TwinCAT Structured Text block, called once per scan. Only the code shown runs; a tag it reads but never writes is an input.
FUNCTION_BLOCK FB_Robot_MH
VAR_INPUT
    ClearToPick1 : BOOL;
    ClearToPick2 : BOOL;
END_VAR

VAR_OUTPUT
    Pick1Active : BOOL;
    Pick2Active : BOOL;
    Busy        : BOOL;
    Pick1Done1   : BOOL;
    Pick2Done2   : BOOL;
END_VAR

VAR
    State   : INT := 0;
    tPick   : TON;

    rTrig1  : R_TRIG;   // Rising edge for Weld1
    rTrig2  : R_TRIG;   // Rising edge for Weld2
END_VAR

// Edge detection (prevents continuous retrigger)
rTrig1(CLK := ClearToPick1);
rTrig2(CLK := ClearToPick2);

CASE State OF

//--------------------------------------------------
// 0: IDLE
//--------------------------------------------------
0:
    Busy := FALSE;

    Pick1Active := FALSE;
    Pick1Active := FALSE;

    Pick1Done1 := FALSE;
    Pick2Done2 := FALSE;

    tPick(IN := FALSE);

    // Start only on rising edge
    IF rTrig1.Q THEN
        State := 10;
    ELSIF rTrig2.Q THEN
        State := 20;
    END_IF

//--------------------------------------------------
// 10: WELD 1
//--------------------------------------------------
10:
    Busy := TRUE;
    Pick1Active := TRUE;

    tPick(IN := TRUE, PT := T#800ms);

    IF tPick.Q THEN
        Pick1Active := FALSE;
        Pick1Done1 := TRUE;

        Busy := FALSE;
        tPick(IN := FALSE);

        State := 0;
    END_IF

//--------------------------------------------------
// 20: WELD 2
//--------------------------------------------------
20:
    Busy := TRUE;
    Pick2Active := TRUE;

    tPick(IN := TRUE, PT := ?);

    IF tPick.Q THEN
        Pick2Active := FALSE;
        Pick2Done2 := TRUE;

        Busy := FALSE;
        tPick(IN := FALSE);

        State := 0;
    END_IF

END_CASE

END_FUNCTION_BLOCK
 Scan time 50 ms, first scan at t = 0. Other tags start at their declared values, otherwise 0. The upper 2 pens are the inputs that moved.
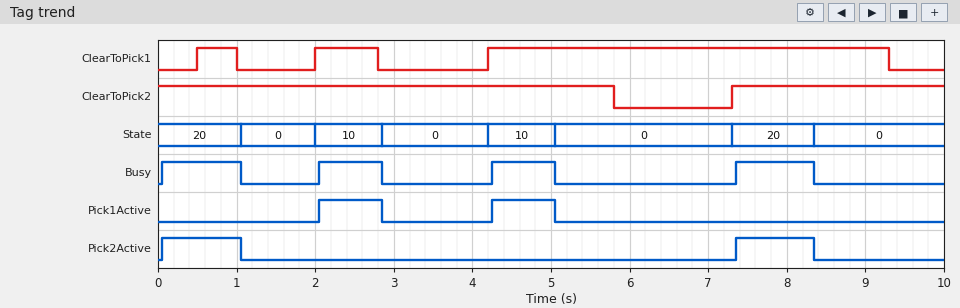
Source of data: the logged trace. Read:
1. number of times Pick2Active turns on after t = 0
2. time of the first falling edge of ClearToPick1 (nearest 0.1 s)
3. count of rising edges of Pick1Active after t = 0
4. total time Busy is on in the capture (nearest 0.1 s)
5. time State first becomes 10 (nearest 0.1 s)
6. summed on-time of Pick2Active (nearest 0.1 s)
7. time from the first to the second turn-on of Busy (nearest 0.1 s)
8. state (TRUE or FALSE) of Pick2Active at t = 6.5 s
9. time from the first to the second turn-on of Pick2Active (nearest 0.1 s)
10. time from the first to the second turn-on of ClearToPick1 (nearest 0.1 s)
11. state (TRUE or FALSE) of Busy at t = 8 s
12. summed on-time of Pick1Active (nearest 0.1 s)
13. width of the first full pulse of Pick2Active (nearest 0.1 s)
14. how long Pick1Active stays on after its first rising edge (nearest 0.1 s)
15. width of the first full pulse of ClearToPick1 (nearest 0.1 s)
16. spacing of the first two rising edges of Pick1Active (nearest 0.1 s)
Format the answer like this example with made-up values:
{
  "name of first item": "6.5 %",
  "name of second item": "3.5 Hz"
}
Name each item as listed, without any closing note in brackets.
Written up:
{
  "number of times Pick2Active turns on after t = 0": "2",
  "time of the first falling edge of ClearToPick1": "1.0 s",
  "count of rising edges of Pick1Active after t = 0": "2",
  "total time Busy is on in the capture": "3.6 s",
  "time State first becomes 10": "2.0 s",
  "summed on-time of Pick2Active": "2.0 s",
  "time from the first to the second turn-on of Busy": "2.0 s",
  "state (TRUE or FALSE) of Pick2Active at t = 6.5 s": "FALSE",
  "time from the first to the second turn-on of Pick2Active": "7.3 s",
  "time from the first to the second turn-on of ClearToPick1": "1.5 s",
  "state (TRUE or FALSE) of Busy at t = 8 s": "TRUE",
  "summed on-time of Pick1Active": "1.6 s",
  "width of the first full pulse of Pick2Active": "1.0 s",
  "how long Pick1Active stays on after its first rising edge": "0.8 s",
  "width of the first full pulse of ClearToPick1": "0.5 s",
  "spacing of the first two rising edges of Pick1Active": "2.2 s"
}
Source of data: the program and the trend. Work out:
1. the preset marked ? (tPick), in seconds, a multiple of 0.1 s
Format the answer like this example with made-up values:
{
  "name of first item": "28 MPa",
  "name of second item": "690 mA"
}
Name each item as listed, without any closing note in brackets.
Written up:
{
  "the preset marked ? (tPick), in seconds, a multiple of 0.1 s": "1.0 s"
}
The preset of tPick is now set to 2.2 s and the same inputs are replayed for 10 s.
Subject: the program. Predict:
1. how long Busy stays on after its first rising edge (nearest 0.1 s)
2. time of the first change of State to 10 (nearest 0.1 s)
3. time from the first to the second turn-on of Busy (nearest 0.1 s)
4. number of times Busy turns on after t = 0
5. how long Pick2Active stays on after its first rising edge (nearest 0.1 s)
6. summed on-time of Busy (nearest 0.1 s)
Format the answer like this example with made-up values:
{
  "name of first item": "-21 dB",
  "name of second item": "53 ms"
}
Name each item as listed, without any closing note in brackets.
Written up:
{
  "how long Busy stays on after its first rising edge": "2.2 s",
  "time of the first change of State to 10": "4.2 s",
  "time from the first to the second turn-on of Busy": "4.2 s",
  "number of times Busy turns on after t = 0": "3",
  "how long Pick2Active stays on after its first rising edge": "2.2 s",
  "summed on-time of Busy": "5.2 s"
}
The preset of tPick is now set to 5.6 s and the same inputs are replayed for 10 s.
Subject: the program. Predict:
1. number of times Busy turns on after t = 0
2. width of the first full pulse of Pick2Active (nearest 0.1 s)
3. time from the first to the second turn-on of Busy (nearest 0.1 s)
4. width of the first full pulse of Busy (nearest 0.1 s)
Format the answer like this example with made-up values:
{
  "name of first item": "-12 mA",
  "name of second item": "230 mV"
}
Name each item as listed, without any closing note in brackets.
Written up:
{
  "number of times Busy turns on after t = 0": "2",
  "width of the first full pulse of Pick2Active": "5.6 s",
  "time from the first to the second turn-on of Busy": "7.3 s",
  "width of the first full pulse of Busy": "5.6 s"
}
